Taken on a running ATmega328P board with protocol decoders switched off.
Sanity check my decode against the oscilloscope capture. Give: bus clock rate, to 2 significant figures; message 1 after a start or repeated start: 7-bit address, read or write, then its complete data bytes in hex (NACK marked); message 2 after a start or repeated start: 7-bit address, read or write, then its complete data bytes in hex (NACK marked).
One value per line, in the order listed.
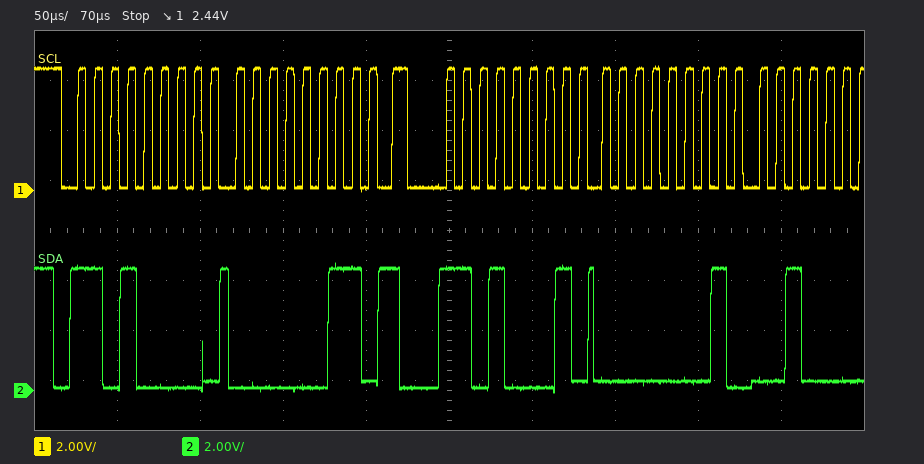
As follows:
100 kHz
0x68 write: 03
0x68 read: 01
